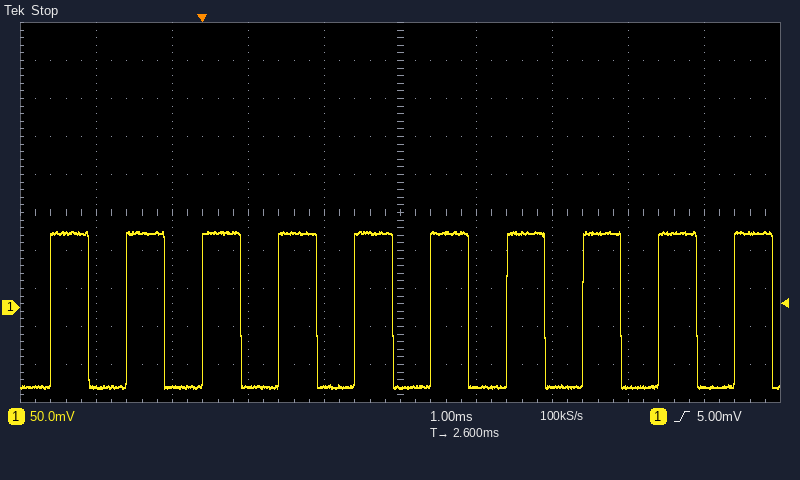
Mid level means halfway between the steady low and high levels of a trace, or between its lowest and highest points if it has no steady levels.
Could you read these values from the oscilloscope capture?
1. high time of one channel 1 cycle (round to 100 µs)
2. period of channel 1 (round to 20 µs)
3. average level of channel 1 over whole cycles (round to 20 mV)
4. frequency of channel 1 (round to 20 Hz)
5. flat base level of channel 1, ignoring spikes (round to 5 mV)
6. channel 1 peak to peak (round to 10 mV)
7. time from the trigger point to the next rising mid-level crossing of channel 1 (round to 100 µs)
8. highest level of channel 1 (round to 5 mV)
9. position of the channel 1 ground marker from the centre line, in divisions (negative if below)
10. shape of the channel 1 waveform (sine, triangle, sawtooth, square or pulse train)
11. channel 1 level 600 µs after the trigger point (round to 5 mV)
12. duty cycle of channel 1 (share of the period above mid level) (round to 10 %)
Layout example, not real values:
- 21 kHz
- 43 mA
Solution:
- 500 µs
- 1.00 ms
- 0 mV
- 1.00 kHz
- -105 mV
- 210 mV
- 1.0 ms
- 100 mV
- -2.5 div
- square
- -105 mV
- 50 %
